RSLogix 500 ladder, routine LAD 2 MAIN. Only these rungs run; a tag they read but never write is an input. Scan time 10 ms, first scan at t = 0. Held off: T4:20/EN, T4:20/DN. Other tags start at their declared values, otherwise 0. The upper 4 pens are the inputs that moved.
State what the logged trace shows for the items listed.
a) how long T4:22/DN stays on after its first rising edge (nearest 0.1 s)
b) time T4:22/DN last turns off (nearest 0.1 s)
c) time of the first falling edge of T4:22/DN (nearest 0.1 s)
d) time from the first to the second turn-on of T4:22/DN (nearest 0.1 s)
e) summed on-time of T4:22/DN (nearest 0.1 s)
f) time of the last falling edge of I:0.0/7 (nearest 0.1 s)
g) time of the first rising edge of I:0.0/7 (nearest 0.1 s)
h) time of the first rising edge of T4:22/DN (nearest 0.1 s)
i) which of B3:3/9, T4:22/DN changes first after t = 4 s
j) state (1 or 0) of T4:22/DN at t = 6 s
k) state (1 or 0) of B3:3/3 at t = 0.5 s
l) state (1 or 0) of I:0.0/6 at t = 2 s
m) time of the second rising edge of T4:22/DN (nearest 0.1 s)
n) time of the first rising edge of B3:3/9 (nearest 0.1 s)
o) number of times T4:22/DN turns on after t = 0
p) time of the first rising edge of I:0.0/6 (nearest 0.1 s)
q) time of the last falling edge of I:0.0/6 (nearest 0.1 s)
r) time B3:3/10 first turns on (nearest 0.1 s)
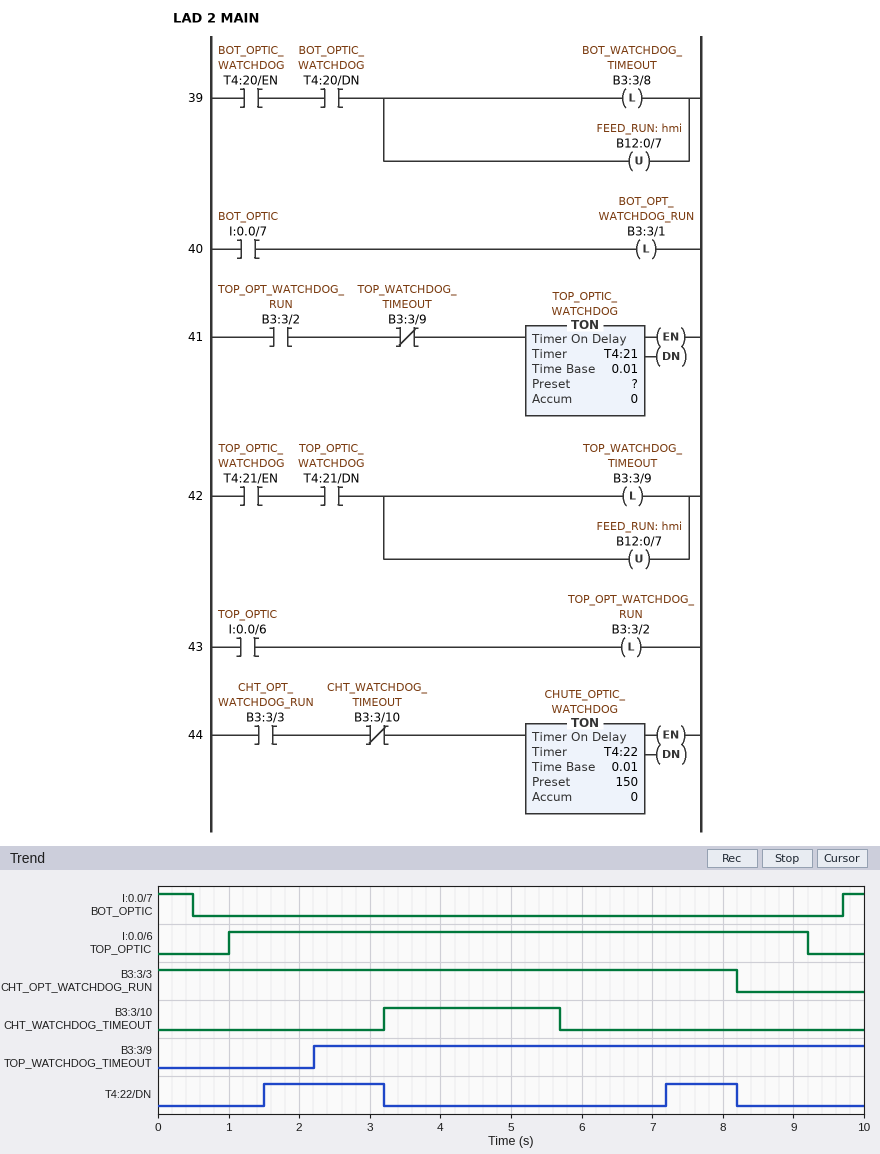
1.7 s
8.2 s
3.2 s
5.7 s
2.7 s
0.5 s
9.7 s
1.5 s
T4:22/DN
0
1
1
7.2 s
2.2 s
2
1.0 s
9.2 s
3.2 s
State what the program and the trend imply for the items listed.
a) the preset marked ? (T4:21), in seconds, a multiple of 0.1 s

1.2 s
